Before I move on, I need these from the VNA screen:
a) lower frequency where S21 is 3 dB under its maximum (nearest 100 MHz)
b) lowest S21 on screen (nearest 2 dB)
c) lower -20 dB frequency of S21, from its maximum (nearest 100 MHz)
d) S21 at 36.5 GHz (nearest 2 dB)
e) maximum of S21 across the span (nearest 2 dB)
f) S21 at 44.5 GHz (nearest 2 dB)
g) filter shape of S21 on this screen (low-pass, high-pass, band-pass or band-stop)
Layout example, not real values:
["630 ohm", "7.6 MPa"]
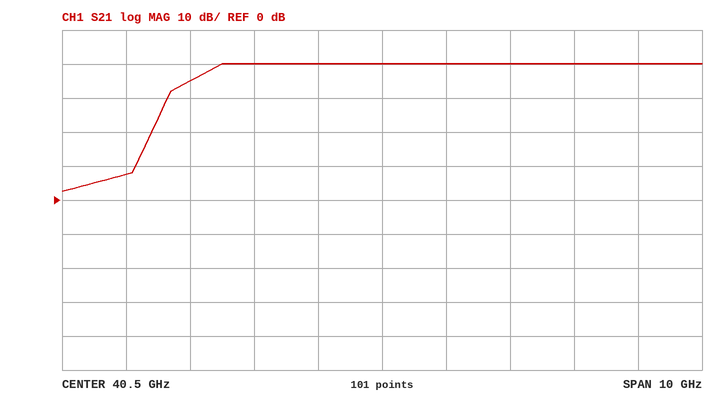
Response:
["37.7 GHz", "2 dB", "36.9 GHz", "8 dB", "40 dB", "40 dB", "high-pass"]
